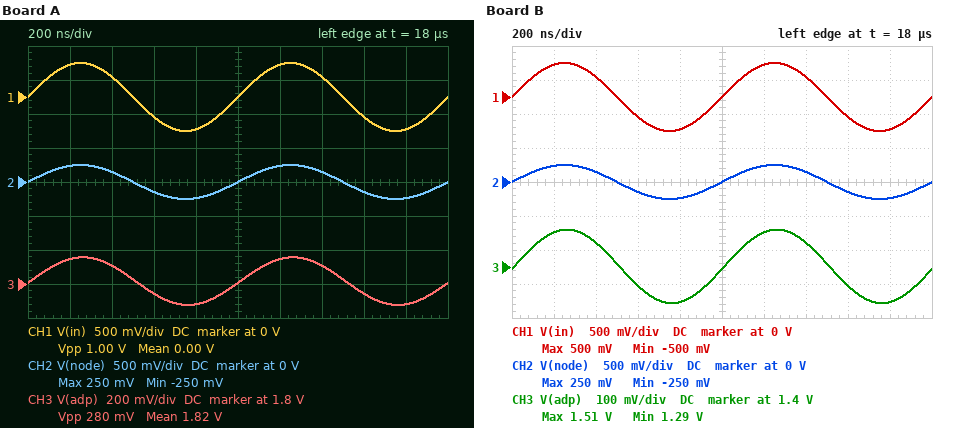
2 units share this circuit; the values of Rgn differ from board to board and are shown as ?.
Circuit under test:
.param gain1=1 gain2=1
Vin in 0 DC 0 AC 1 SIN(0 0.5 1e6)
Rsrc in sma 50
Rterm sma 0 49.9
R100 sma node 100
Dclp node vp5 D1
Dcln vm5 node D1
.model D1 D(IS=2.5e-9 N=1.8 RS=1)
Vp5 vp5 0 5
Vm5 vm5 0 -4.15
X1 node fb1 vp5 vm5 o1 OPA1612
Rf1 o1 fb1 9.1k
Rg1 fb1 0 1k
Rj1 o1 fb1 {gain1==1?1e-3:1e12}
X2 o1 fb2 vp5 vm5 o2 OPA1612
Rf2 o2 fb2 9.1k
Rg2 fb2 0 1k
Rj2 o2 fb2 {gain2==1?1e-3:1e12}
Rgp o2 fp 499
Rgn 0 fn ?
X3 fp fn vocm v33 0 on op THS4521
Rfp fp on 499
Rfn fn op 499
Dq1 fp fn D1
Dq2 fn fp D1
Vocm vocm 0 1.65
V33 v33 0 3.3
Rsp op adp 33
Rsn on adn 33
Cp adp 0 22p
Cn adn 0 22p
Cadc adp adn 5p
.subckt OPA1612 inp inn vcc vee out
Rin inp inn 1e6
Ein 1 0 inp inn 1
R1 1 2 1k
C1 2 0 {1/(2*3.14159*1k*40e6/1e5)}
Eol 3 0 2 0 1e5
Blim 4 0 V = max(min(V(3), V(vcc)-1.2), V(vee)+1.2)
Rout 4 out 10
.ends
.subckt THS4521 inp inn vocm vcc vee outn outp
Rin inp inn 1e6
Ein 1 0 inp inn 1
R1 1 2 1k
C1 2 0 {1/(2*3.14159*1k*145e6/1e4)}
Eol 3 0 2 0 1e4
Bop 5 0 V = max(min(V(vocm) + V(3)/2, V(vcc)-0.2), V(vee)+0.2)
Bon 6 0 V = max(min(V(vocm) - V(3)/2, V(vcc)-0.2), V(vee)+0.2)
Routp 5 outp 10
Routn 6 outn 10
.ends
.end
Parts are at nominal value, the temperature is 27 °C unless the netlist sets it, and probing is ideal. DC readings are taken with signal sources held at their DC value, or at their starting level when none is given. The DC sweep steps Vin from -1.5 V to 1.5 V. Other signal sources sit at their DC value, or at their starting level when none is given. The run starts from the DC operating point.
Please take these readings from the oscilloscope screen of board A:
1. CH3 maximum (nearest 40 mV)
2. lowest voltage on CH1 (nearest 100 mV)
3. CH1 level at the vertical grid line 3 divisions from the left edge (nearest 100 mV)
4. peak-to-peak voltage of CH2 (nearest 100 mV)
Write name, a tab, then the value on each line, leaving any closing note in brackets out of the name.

CH3 maximum	1.96 V
lowest voltage on CH1	-500 mV
CH1 level at the vertical grid line 3 divisions from the left edge	-300 mV
peak-to-peak voltage of CH2	500 mV
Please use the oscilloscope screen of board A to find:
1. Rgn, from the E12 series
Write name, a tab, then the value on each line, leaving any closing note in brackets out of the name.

Rgn, from the E12 series	330 Ω
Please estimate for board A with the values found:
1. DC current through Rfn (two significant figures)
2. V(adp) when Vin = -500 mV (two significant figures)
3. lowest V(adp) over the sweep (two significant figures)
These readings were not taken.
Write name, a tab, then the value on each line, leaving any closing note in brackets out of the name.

DC current through Rfn	2.2 mA
V(adp) when Vin = -500 mV	1.7 V
lowest V(adp) over the sweep	1.4 V
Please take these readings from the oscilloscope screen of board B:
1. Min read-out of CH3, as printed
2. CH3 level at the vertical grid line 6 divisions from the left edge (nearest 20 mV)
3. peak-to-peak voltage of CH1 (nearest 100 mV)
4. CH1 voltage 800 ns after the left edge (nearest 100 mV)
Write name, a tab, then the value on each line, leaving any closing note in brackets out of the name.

Min read-out of CH3, as printed	1.29 V
CH3 level at the vertical grid line 6 divisions from the left edge	1.50 V
peak-to-peak voltage of CH1	1.0 V
CH1 voltage 800 ns after the left edge	-500 mV
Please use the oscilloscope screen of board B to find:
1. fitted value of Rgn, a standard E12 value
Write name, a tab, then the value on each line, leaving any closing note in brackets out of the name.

fitted value of Rgn, a standard E12 value	1 kΩ
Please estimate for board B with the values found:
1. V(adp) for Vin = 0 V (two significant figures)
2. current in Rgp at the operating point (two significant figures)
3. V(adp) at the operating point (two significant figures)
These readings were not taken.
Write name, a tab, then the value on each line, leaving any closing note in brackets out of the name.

V(adp) for Vin = 0 V	1.4 V
current in Rgp at the operating point	1.9 mA
V(adp) at the operating point	1.4 V
